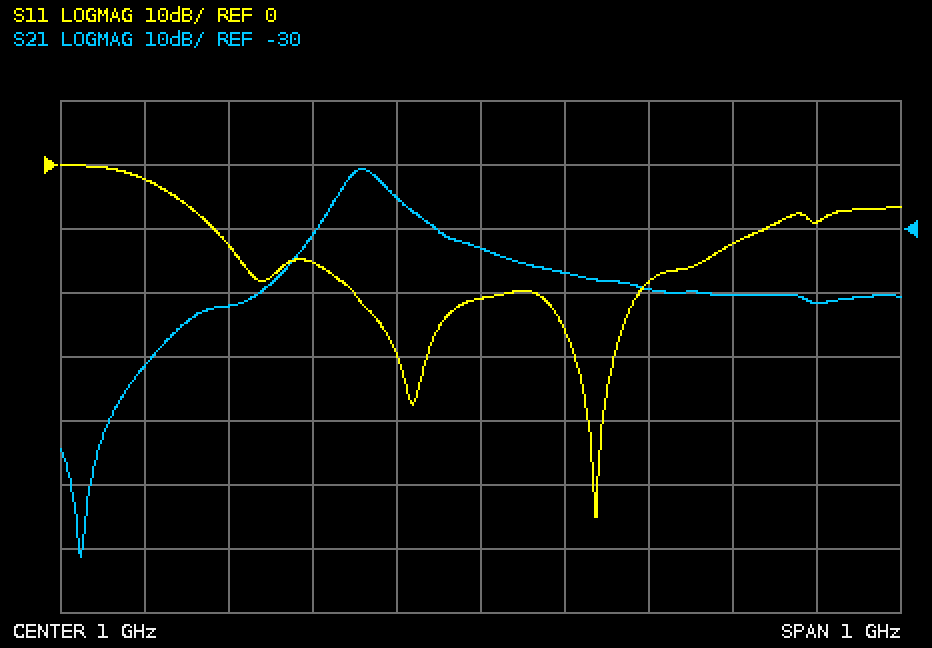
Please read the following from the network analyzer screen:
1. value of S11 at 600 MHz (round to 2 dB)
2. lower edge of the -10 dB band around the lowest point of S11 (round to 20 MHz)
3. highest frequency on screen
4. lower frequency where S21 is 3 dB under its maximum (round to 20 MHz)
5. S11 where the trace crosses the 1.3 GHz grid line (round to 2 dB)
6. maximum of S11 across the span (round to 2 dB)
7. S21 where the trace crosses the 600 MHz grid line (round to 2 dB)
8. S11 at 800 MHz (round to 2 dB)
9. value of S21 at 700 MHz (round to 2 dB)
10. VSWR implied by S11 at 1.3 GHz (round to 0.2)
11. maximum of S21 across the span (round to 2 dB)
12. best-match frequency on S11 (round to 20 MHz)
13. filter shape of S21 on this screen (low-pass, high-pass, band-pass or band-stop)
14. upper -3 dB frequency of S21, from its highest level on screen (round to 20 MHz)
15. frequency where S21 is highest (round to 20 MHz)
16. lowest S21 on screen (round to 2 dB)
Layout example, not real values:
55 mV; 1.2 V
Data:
-2 dB; 680 MHz; 1.5 GHz; 840 MHz; -12 dB; 0 dB; -52 dB; -16 dB; -42 dB; 1.6; -20 dB; 1.14 GHz; band-pass; 880 MHz; 860 MHz; -82 dB
